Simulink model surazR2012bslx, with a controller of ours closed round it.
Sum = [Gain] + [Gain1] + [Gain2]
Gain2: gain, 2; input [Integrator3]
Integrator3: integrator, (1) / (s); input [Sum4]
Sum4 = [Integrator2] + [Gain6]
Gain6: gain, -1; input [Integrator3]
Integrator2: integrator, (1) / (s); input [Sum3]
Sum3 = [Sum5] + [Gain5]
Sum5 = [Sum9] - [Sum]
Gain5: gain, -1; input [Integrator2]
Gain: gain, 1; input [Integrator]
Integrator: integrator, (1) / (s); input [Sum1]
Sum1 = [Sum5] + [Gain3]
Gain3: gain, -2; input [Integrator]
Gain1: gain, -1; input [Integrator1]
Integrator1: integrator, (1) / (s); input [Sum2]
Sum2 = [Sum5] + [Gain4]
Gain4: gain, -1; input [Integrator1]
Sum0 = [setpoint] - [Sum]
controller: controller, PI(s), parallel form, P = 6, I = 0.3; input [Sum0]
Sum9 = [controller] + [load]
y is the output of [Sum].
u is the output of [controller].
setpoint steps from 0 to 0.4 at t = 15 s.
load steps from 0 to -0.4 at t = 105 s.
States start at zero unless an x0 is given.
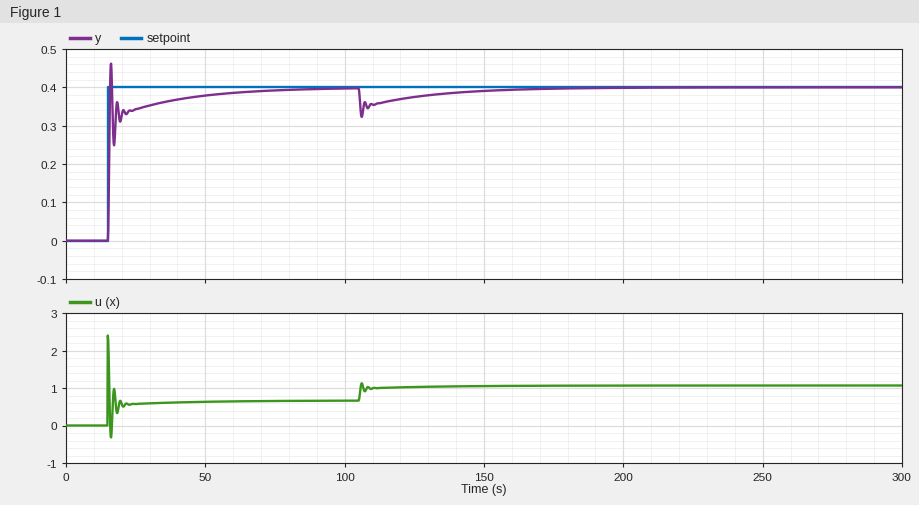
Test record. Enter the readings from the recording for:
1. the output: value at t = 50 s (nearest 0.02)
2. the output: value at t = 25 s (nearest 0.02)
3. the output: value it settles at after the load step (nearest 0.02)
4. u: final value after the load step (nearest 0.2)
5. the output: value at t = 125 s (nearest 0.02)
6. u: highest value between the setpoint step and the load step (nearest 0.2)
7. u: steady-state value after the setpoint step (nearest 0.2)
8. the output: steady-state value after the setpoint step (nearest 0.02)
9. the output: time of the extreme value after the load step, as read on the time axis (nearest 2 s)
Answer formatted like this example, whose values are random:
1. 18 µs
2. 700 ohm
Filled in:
1. 0.38
2. 0.34
3. 0.40
4. 1.0
5. 0.38
6. 2.4
7. 0.6
8. 0.40
9. 106 s
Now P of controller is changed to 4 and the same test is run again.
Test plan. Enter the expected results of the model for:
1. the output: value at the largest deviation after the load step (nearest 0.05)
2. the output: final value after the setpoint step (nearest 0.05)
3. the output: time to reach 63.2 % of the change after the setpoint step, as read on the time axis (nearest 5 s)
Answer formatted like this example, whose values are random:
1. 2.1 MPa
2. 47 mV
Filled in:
1. 0.30
2. 0.40
3. 15 s
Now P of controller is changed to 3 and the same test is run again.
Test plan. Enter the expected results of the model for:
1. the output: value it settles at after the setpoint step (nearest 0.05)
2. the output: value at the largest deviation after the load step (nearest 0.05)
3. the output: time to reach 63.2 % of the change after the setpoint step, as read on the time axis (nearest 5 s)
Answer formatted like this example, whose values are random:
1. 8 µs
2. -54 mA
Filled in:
1. 0.40
2. 0.30
3. 15 s
